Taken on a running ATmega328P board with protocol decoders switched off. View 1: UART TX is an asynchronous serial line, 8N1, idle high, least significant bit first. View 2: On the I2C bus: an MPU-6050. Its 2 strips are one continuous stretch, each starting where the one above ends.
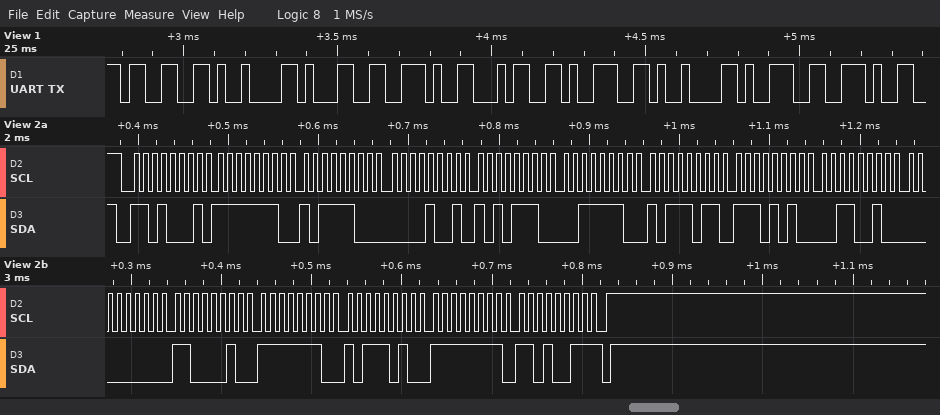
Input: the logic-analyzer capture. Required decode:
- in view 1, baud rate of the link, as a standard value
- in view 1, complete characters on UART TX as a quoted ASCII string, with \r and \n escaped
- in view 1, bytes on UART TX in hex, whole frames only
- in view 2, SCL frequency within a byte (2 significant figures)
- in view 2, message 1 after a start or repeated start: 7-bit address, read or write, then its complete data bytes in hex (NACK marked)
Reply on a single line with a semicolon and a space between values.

38400 baud; "3\t1.49\t9."; 33 09 31 2E 34 39 09 39 2E; 100 kHz; 0x68 read: FE BC 09 AE 3E BB EA 32 00 C2 FE BA FF D3 NACK
